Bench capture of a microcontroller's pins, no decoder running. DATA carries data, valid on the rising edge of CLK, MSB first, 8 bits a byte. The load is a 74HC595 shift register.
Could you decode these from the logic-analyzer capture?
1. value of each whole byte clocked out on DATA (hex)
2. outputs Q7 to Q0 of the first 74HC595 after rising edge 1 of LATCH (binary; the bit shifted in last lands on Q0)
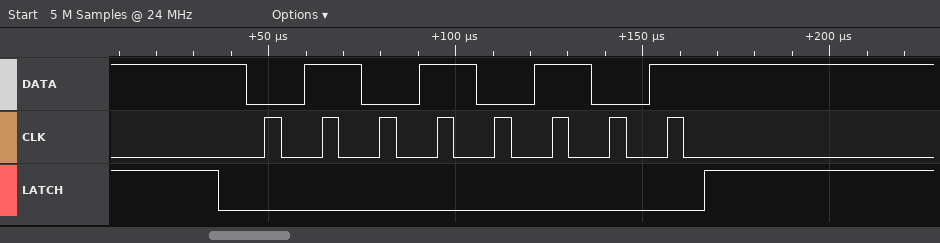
0x55
01010101
